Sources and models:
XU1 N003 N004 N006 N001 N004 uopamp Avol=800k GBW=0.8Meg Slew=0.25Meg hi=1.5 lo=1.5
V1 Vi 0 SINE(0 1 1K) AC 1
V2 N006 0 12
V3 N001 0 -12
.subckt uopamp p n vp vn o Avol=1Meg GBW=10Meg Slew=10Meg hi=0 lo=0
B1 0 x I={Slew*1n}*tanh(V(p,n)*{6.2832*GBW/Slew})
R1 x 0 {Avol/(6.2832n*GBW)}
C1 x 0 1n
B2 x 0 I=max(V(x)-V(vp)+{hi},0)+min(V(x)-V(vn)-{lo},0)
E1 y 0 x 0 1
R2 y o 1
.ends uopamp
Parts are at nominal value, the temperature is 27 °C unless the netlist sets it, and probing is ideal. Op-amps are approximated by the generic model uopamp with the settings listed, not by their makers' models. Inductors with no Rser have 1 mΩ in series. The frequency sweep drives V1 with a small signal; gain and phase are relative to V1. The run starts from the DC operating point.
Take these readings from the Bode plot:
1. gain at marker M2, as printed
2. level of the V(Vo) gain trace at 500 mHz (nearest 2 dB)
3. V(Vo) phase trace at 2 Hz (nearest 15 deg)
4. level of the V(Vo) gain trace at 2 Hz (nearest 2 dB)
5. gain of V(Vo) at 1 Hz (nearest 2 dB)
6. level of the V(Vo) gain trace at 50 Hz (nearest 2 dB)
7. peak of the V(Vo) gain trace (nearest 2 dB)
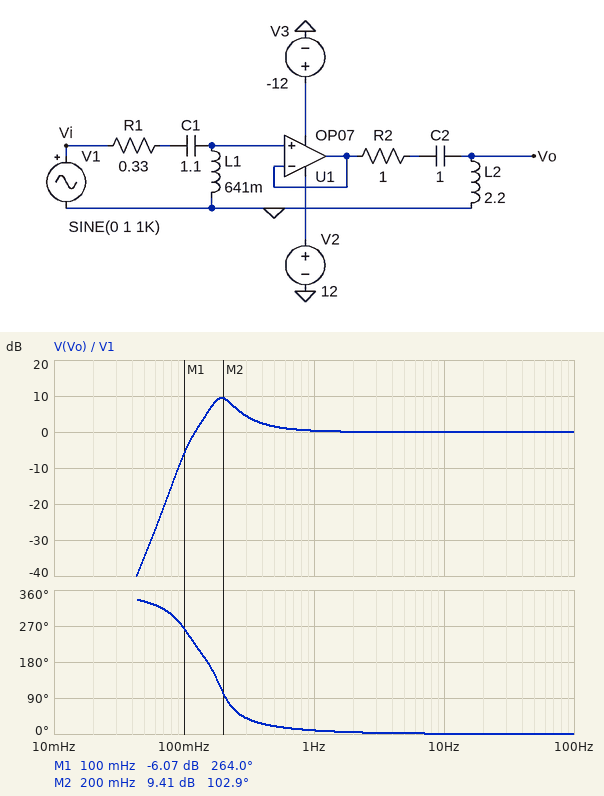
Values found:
9.41 dB
2 dB
0 deg
0 dB
0 dB
0 dB
10 dB
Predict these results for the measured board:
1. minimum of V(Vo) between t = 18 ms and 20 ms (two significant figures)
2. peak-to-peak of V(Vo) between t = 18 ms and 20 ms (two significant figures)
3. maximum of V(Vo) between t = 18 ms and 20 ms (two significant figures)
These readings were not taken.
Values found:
-1.0 V
2.0 V
1.0 V
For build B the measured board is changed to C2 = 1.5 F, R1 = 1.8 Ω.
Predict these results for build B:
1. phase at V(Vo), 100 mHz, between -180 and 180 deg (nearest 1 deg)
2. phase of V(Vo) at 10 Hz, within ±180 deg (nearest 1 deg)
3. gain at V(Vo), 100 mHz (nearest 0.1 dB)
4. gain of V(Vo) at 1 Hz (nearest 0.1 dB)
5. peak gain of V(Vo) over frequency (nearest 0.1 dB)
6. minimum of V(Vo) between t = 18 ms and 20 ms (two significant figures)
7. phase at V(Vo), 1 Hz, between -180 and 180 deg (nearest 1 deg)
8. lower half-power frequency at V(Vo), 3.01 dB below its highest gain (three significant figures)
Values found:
-168 deg
3 deg
-11.9 dB
-0.5 dB
0 dB
-1.0 V
29 deg
344 mHz
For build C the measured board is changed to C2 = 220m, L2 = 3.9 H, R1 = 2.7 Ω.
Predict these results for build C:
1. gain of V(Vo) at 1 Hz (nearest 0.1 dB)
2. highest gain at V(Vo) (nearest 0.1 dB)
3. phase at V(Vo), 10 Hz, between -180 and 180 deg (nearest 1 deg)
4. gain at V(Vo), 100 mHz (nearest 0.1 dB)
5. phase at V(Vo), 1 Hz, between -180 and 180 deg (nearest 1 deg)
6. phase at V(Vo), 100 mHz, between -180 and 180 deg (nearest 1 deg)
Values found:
-1.1 dB
0.9 dB
4 deg
-23.1 dB
37 deg
-81 deg
